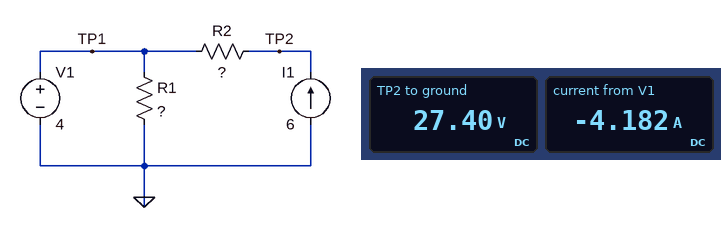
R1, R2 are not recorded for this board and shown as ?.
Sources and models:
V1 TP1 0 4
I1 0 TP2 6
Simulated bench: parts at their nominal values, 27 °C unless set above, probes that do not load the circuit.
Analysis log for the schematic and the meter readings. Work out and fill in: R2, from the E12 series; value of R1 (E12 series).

3.9 Ω
2.2 Ω
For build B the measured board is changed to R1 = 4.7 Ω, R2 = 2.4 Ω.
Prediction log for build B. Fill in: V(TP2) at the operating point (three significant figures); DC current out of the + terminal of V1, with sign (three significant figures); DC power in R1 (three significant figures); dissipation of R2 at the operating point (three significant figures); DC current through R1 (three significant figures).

18.4 V
-5.15 A
3.40 W
86.4 W
851 mA
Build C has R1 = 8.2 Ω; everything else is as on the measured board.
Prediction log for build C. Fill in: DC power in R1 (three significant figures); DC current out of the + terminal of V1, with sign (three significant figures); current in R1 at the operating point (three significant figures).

1.95 W
-5.51 A
488 mA
